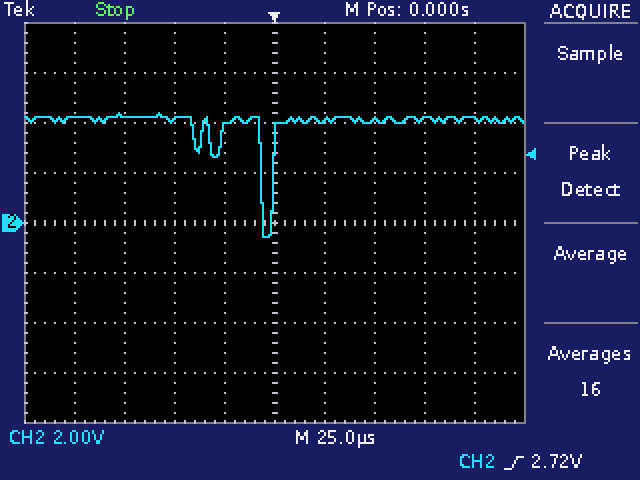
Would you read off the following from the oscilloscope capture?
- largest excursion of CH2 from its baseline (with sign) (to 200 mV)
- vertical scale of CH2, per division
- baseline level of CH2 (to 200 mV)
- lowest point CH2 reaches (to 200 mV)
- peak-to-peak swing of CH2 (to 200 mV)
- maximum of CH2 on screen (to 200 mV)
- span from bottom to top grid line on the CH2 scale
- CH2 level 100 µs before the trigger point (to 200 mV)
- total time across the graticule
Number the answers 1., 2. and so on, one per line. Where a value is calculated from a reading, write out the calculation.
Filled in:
1. -600 mV − (4.2 V) = -4.8 V
2. 2 V
3. 4.2 V
4. -600 mV
5. 4.4 V − (-600 mV) = 5.0 V
6. 4.4 V
7. 16 V
8. 4.2 V
9. 250 µs
